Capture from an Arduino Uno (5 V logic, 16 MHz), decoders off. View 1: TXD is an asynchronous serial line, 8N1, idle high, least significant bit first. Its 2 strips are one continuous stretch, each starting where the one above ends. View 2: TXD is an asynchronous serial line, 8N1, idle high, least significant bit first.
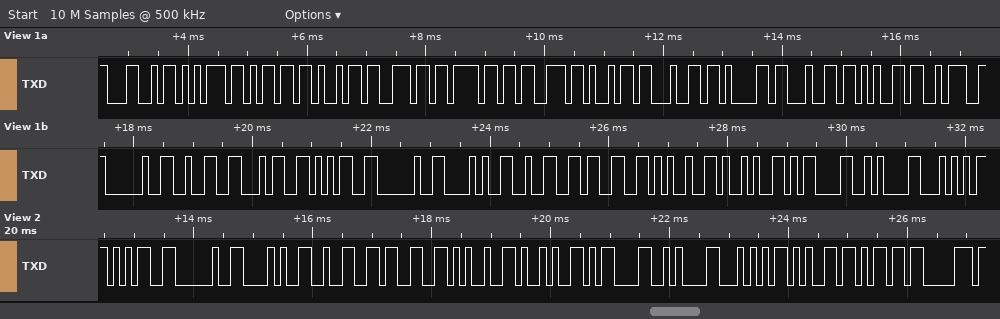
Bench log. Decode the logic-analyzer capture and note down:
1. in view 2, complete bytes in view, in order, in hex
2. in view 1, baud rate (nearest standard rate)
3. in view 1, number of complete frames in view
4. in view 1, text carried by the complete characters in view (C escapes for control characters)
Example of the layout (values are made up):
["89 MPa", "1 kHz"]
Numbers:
["35 20 28 32 33 25 29 0D 0A 54 65 6D 70", "9600 baud", "26", "\"Luminosidade: 245 (23%)\\r\\nT\""]
